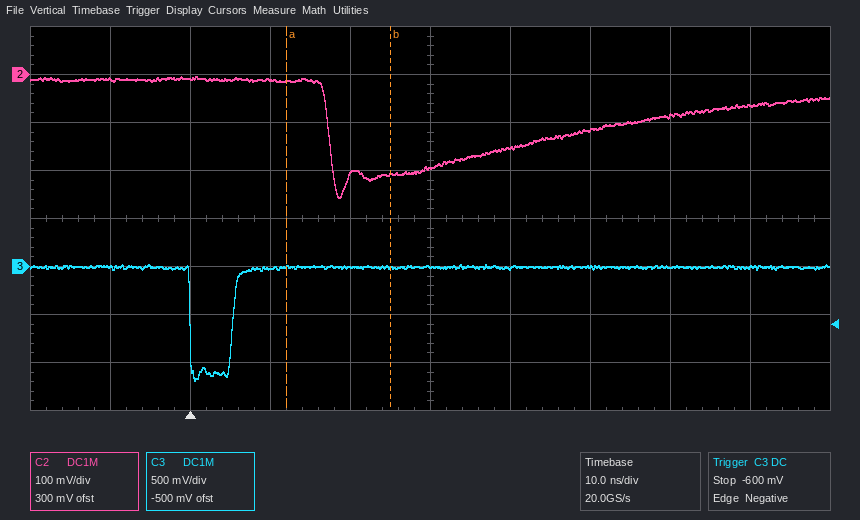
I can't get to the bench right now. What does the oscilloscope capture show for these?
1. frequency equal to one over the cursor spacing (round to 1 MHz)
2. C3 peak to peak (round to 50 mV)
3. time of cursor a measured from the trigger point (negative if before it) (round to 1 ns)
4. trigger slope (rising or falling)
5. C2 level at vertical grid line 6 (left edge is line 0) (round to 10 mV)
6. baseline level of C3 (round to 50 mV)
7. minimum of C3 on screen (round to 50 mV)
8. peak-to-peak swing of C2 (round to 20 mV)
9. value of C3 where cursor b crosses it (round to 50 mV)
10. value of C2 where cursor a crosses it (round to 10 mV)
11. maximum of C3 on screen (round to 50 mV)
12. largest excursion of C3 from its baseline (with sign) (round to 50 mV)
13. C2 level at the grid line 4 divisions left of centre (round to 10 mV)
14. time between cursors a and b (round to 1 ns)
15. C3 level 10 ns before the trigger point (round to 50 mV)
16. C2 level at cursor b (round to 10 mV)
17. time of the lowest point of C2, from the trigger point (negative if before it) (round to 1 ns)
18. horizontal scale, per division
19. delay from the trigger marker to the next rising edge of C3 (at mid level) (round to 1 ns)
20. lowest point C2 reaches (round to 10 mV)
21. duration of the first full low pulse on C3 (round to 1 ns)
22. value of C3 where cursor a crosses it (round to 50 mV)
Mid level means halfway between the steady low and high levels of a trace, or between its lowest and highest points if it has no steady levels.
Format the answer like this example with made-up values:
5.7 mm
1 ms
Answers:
77 MHz
1.20 V
+12 ns
falling
-150 mV
0 mV
-1.20 V
260 mV
0 mV
-10 mV
0 mV
-1.20 V
-10 mV
13 ns
0 mV
-210 mV
+19 ns
10 ns
5 ns
-260 mV
5 ns
0 mV
